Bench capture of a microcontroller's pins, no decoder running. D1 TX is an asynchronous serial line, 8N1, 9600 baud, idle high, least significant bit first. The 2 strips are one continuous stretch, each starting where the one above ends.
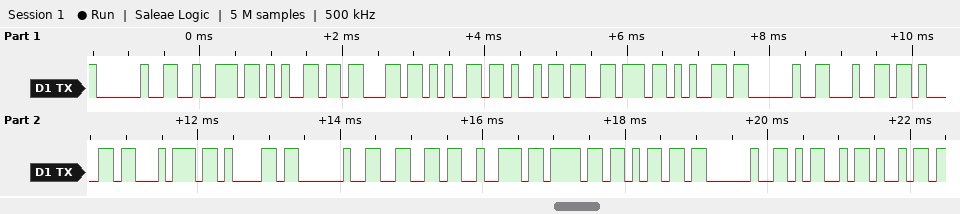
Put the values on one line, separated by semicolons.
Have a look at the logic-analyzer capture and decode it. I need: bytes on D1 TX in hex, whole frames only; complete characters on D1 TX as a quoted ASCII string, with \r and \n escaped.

20 72 65 63 65 69 76 65 20 64 61 74 61 20 66 72 6F 6D 20 4D 69; " receive data from Mi"
